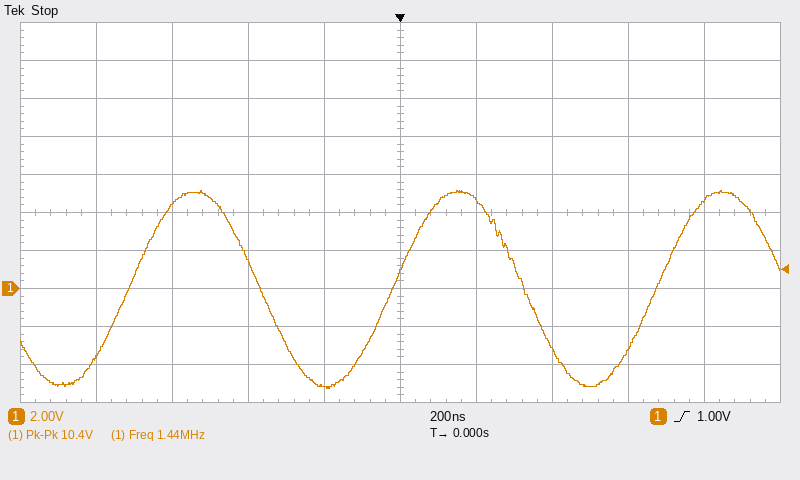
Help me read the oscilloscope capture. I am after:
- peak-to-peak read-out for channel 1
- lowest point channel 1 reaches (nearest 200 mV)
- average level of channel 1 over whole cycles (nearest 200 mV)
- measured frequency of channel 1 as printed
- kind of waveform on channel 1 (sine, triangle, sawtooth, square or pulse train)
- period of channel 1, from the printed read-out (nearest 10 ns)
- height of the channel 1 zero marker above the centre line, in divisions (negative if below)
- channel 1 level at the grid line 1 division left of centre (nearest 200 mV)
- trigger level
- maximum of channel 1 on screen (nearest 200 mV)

10.4 V
-5.2 V
0.0 V
1.44 MHz
sine
690 ns
-2.0 div
-5.2 V
1.00 V
5.2 V
